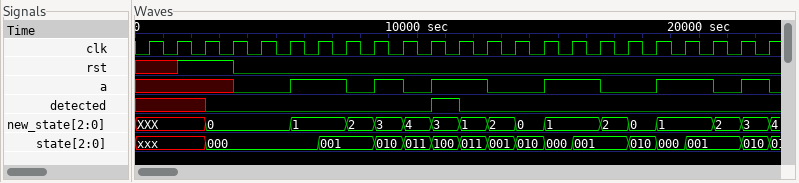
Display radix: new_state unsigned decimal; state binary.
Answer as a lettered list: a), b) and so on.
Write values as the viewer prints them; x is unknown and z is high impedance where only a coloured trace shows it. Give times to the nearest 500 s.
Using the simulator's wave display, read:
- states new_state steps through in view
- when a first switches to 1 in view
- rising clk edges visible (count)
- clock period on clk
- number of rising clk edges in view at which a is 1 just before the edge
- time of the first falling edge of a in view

a) XXX, 0, 1, 2, 3, 4, 3, 1, 2, 0, 1, 2, 0, 1, 2, 3, 4
b) 5500 s
c) 23
d) 1000 s
e) 10
f) 7500 s
